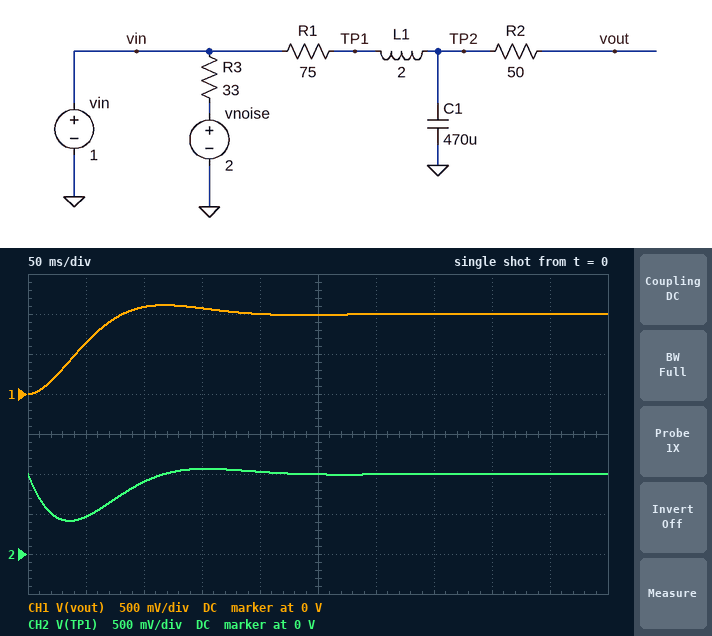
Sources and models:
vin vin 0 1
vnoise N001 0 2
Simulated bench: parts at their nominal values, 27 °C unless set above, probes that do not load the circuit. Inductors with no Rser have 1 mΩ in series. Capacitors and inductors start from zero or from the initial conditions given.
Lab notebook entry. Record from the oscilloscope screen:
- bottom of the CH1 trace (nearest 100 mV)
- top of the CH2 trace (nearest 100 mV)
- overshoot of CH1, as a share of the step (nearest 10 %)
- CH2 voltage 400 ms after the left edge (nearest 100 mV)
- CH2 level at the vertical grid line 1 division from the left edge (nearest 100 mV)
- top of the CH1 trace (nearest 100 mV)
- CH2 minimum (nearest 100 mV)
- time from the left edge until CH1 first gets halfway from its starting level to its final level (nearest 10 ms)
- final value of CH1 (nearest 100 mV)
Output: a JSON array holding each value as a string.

["0 V", "1.1 V", "10 %", "1.0 V", "500 mV", "1.1 V", "400 mV", "40 ms", "1.0 V"]
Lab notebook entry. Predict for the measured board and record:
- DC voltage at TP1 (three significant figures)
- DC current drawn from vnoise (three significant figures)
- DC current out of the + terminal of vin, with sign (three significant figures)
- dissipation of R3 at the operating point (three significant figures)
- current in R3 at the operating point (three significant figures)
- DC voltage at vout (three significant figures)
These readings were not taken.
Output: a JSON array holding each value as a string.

["1.00 V", "30.3 mA", "-30.3 mA", "30.3 mW", "30.3 mA", "1.00 V"]
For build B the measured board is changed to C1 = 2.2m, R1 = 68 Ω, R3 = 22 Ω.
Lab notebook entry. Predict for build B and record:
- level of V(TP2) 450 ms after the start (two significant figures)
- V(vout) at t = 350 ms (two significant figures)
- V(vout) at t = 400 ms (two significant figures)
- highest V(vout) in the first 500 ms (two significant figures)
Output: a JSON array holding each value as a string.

["970 mV", "940 mV", "960 mV", "980 mV"]
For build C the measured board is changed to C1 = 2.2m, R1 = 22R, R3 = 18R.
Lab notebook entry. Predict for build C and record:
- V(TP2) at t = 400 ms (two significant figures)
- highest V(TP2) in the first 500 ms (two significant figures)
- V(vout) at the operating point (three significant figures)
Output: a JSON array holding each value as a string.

["940 mV", "1.3 V", "1.00 V"]
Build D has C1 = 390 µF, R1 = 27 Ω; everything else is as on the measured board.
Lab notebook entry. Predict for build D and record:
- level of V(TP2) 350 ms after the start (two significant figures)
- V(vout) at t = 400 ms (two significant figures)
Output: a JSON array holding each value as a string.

["910 mV", "980 mV"]
